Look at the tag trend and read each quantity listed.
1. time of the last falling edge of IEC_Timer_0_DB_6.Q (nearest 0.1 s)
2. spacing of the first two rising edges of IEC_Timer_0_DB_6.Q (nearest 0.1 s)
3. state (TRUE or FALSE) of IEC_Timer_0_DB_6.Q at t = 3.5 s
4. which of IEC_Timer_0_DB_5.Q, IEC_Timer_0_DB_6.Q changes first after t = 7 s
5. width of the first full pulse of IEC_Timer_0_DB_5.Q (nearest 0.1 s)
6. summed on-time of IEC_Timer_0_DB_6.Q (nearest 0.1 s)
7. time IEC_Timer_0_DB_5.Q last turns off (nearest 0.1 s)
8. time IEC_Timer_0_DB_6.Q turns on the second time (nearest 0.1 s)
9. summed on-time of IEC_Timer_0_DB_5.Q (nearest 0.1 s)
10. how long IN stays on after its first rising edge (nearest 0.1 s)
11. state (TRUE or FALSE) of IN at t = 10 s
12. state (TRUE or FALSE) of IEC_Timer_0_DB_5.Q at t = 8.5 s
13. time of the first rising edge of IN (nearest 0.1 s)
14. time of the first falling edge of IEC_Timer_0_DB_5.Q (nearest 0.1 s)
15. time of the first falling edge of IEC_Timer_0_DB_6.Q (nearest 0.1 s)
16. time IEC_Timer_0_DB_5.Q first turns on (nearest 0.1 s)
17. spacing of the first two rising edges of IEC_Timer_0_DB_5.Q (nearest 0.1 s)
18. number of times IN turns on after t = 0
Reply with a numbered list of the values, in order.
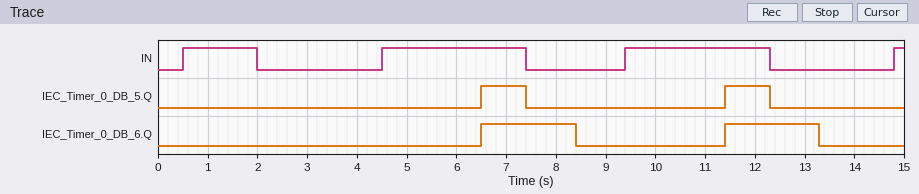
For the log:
1. 13.3 s
2. 4.9 s
3. FALSE
4. IEC_Timer_0_DB_5.Q
5. 0.9 s
6. 3.8 s
7. 12.3 s
8. 11.4 s
9. 1.8 s
10. 1.5 s
11. TRUE
12. FALSE
13. 0.5 s
14. 7.4 s
15. 8.4 s
16. 6.5 s
17. 4.9 s
18. 4
